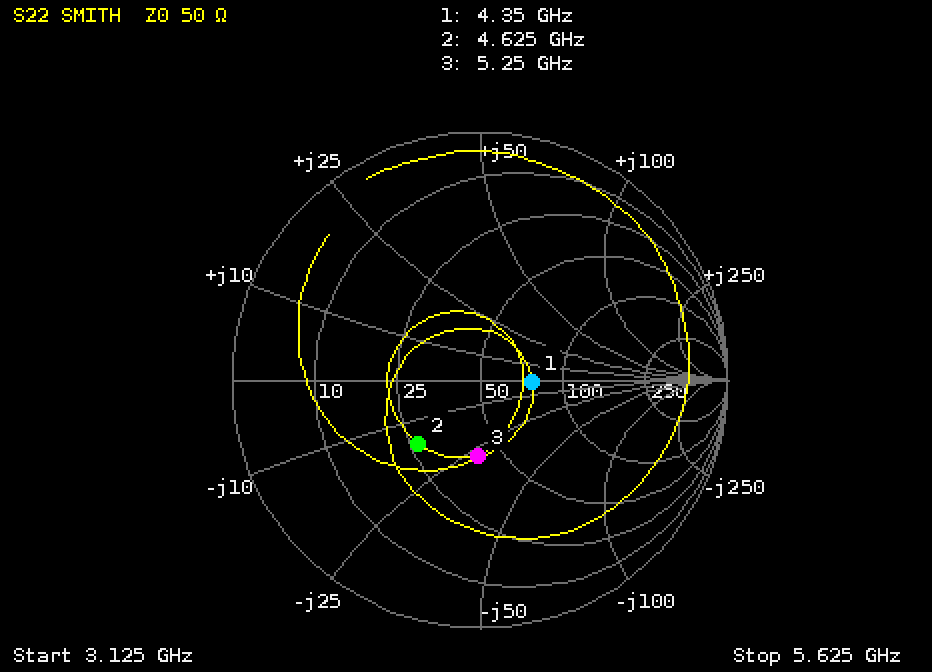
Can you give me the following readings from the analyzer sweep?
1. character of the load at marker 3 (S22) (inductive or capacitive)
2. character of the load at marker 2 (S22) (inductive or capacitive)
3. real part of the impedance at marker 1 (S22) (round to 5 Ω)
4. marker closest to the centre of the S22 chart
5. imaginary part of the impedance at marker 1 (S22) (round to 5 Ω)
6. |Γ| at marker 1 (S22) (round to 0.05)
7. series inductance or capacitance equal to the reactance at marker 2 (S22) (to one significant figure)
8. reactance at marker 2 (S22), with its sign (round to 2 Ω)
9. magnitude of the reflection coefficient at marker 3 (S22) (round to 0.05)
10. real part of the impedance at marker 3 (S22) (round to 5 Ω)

capacitive
capacitive
75 Ω
marker 1
0 Ω
0.20
2 pF
-16 Ω
0.30
40 Ω
